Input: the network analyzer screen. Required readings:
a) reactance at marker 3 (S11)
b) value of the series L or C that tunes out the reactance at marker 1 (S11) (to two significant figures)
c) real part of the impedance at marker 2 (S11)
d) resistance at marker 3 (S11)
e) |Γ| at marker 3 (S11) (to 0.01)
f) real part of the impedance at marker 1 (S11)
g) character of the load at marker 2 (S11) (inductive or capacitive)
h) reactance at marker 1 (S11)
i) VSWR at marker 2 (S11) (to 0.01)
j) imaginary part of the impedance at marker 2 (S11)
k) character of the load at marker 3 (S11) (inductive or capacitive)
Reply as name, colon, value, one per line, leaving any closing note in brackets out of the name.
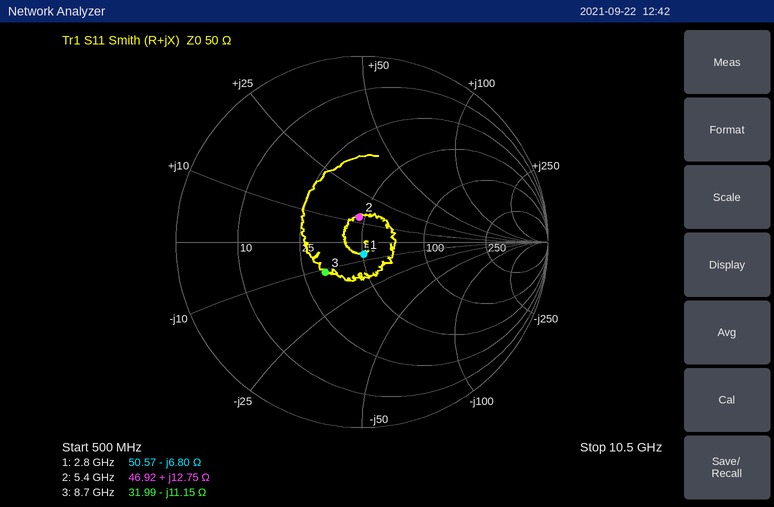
reactance at marker 3: -11.15 Ω
value of the series L or C that tunes out the reactance at marker 1 (S11): 390 pH
real part of the impedance at marker 2: 46.92 Ω
resistance at marker 3: 31.99 Ω
|Γ| at marker 3 (S11): 0.26
real part of the impedance at marker 1: 50.57 Ω
character of the load at marker 2 (S11): inductive
reactance at marker 1: -6.80 Ω
VSWR at marker 2 (S11): 1.31
imaginary part of the impedance at marker 2: +12.75 Ω
character of the load at marker 3 (S11): capacitive
